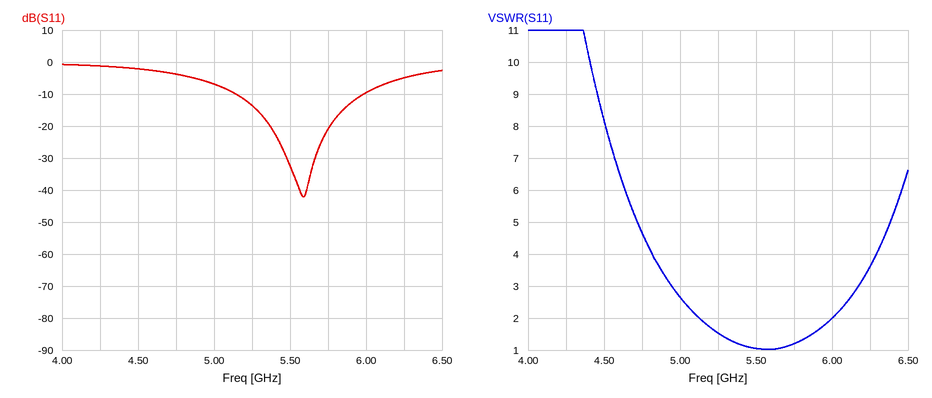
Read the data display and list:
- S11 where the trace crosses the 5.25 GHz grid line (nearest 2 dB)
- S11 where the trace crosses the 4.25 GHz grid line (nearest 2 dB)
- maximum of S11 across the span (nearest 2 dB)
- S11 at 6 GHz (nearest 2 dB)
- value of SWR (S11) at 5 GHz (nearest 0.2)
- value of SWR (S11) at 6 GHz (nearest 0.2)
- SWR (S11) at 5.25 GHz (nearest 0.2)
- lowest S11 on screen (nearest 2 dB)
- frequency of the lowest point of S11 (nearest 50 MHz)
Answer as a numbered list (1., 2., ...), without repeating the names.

1. -14 dB
2. -2 dB
3. 0 dB
4. -10 dB
5. 2.6
6. 2.0
7. 1.6
8. -42 dB
9. 5.60 GHz
